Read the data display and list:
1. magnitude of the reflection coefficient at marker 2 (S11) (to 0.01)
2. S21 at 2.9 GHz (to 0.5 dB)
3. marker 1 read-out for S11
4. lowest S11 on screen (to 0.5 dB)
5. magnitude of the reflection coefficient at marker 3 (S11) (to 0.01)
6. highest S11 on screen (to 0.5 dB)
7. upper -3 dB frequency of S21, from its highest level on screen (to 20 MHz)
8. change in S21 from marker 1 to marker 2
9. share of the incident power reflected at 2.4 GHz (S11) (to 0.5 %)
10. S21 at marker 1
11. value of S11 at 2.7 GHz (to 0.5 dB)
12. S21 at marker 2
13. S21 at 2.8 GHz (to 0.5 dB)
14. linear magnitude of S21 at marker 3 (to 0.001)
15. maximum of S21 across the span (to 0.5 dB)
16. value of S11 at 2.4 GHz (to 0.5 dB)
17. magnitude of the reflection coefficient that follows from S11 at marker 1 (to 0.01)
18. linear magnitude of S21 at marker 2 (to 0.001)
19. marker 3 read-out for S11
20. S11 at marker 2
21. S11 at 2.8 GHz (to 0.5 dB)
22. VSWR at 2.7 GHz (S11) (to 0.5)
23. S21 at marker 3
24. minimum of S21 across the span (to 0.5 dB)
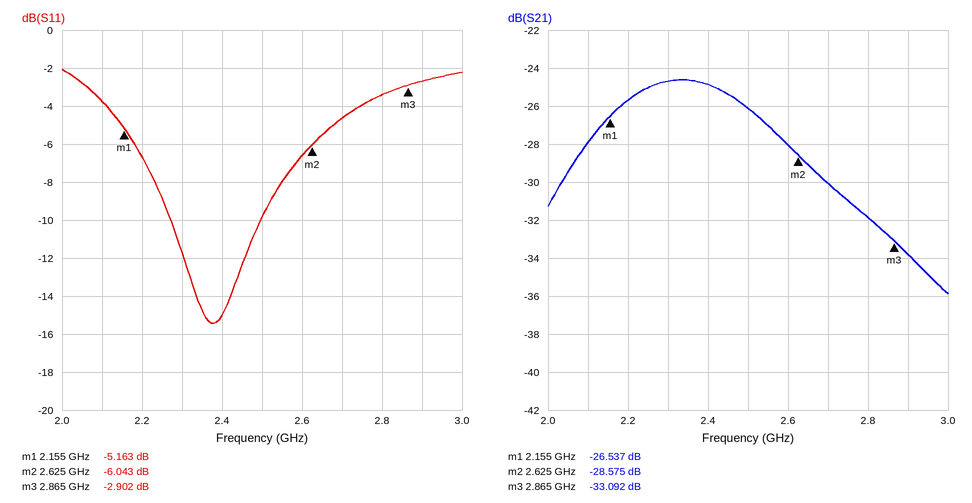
0.50
-34.0 dB
-5.163 dB
-15.5 dB
0.72
-2.0 dB
2.58 GHz
-2.038 dB
3.0 %
-26.537 dB
-4.5 dB
-28.575 dB
-32.0 dB
0.022
-24.5 dB
-15.0 dB
0.55
0.037
-2.902 dB
-6.043 dB
-3.5 dB
4.0
-33.092 dB
-36.0 dB
